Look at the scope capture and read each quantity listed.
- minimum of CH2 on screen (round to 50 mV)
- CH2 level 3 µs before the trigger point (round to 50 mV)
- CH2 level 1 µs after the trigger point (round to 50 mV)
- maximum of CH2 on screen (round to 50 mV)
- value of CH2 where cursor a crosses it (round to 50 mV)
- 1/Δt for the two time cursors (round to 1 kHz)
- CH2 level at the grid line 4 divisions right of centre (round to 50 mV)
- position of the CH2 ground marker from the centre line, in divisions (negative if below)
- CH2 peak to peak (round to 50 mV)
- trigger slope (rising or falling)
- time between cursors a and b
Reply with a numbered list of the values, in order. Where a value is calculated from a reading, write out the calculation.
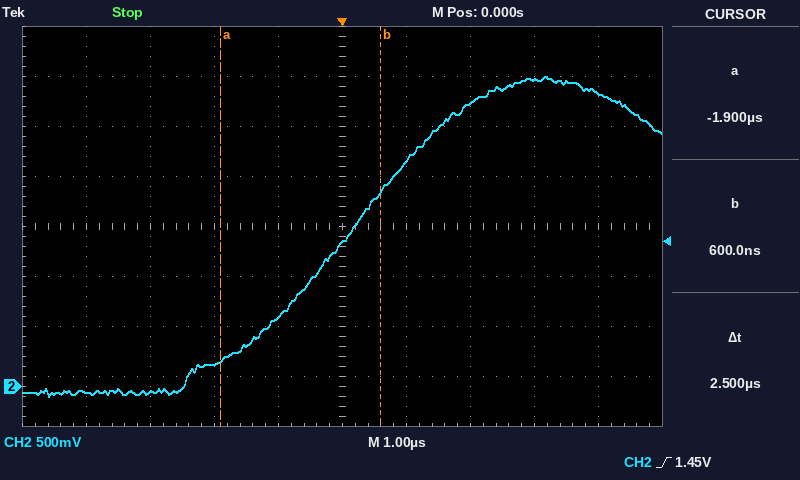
1. -100 mV
2. -50 mV
3. 2.25 V
4. 3.10 V
5. 250 mV
6. 1 / 2.5 µs ≈ 400 kHz
7. 2.95 V
8. -3.2 div
9. 3.10 V − (-100 mV) = 3.20 V
10. rising
11. 2.5 µs
